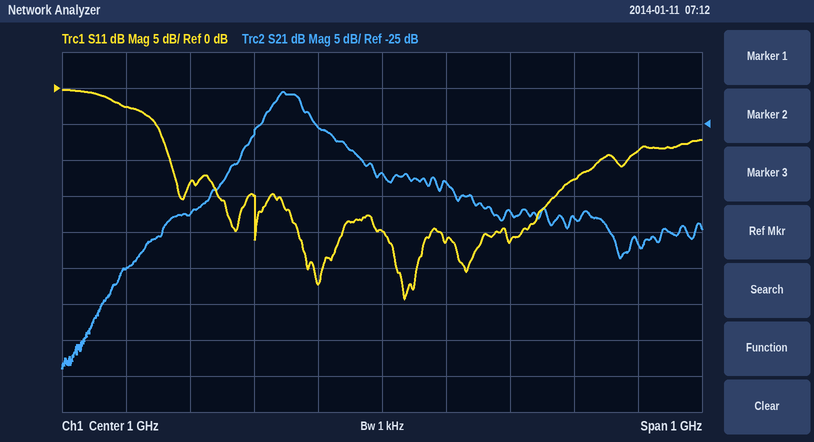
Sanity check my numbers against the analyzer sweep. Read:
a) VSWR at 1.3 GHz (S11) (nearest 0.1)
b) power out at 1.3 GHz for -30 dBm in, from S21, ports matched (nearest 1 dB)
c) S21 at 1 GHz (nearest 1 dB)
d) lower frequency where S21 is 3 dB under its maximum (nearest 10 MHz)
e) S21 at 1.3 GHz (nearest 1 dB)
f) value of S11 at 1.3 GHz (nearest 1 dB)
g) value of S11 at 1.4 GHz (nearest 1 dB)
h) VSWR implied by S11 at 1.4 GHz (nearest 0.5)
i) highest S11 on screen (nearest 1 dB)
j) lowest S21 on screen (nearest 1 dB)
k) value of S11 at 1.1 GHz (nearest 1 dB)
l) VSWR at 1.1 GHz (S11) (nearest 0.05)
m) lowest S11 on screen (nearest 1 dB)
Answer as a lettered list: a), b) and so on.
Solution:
a) 1.6
b) -68 dBm
c) -32 dB
d) 820 MHz
e) -38 dB
f) -13 dB
g) -9 dB
h) 2.0
i) 0 dB
j) -59 dB
k) -21 dB
l) 1.20
m) -29 dB
